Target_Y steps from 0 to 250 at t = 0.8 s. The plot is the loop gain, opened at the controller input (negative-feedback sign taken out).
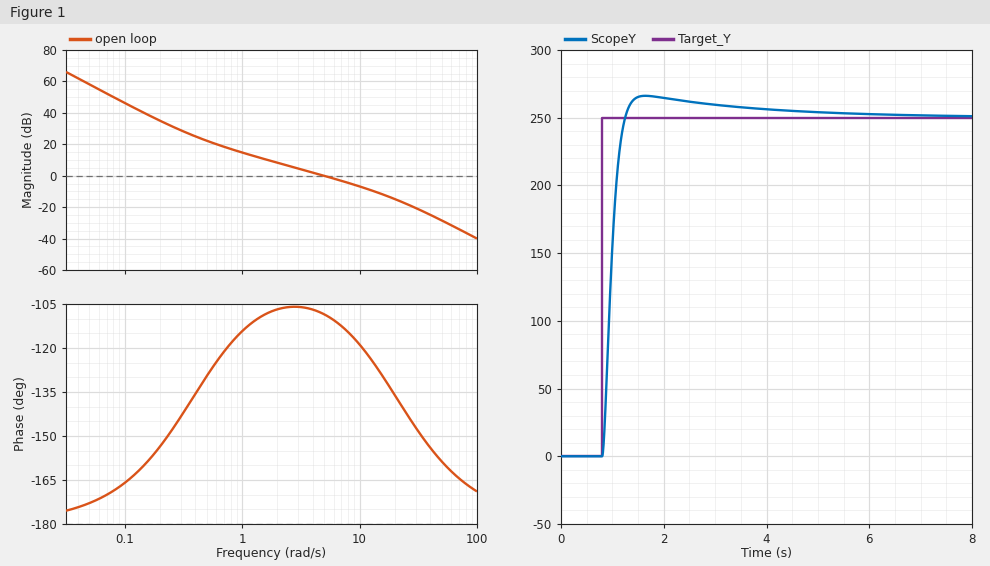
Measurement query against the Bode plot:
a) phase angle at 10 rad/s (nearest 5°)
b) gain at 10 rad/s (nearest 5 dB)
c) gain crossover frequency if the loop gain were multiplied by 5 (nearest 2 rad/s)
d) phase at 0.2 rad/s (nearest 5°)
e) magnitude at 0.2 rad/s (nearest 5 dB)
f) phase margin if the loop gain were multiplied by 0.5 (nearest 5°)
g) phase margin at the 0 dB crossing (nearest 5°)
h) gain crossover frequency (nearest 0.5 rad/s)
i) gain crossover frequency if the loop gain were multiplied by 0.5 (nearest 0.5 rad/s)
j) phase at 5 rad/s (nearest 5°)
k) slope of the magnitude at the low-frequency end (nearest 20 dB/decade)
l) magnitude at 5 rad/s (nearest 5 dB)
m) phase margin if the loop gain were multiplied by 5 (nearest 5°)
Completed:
-120°
-5 dB
18 rad/s
-155°
35 dB
75°
70°
5.0 rad/s
2.5 rad/s
-110°
-40 dB/decade
0 dB
45°
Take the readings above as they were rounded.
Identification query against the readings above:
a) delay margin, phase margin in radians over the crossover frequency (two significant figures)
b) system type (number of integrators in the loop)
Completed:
0.24 s
2
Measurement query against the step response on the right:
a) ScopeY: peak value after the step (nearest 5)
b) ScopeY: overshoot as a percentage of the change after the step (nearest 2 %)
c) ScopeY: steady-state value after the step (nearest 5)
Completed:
265
6 %
250
